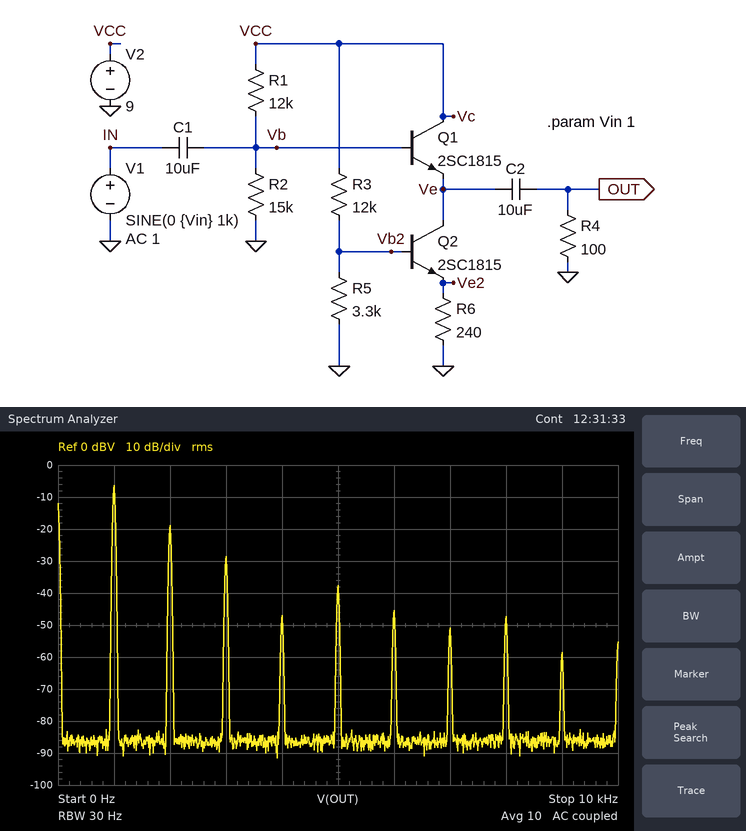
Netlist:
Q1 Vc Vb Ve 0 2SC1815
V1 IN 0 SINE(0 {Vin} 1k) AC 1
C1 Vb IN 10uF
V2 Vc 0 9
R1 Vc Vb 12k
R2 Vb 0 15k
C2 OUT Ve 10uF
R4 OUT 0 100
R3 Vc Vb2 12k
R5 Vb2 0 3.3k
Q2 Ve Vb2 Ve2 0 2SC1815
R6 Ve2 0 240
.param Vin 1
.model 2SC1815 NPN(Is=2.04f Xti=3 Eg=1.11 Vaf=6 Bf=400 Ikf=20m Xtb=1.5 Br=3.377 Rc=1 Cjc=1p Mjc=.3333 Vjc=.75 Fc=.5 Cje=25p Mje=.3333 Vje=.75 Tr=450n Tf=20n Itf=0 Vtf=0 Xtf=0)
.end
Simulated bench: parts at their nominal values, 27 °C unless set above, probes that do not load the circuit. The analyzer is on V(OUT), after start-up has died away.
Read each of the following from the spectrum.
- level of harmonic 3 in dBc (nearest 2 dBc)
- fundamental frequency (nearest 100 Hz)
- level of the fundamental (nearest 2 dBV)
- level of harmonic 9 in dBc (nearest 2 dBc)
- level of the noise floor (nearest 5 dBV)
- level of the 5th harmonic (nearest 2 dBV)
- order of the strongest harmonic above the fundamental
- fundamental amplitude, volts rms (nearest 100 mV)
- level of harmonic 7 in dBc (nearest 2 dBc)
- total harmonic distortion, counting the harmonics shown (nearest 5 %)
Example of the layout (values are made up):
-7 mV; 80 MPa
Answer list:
-22 dBc; 1.0 kHz; -6 dBV; -52 dBc; -85 dBV; -38 dBV; 2; 500 mV; -44 dBc; 25 %
